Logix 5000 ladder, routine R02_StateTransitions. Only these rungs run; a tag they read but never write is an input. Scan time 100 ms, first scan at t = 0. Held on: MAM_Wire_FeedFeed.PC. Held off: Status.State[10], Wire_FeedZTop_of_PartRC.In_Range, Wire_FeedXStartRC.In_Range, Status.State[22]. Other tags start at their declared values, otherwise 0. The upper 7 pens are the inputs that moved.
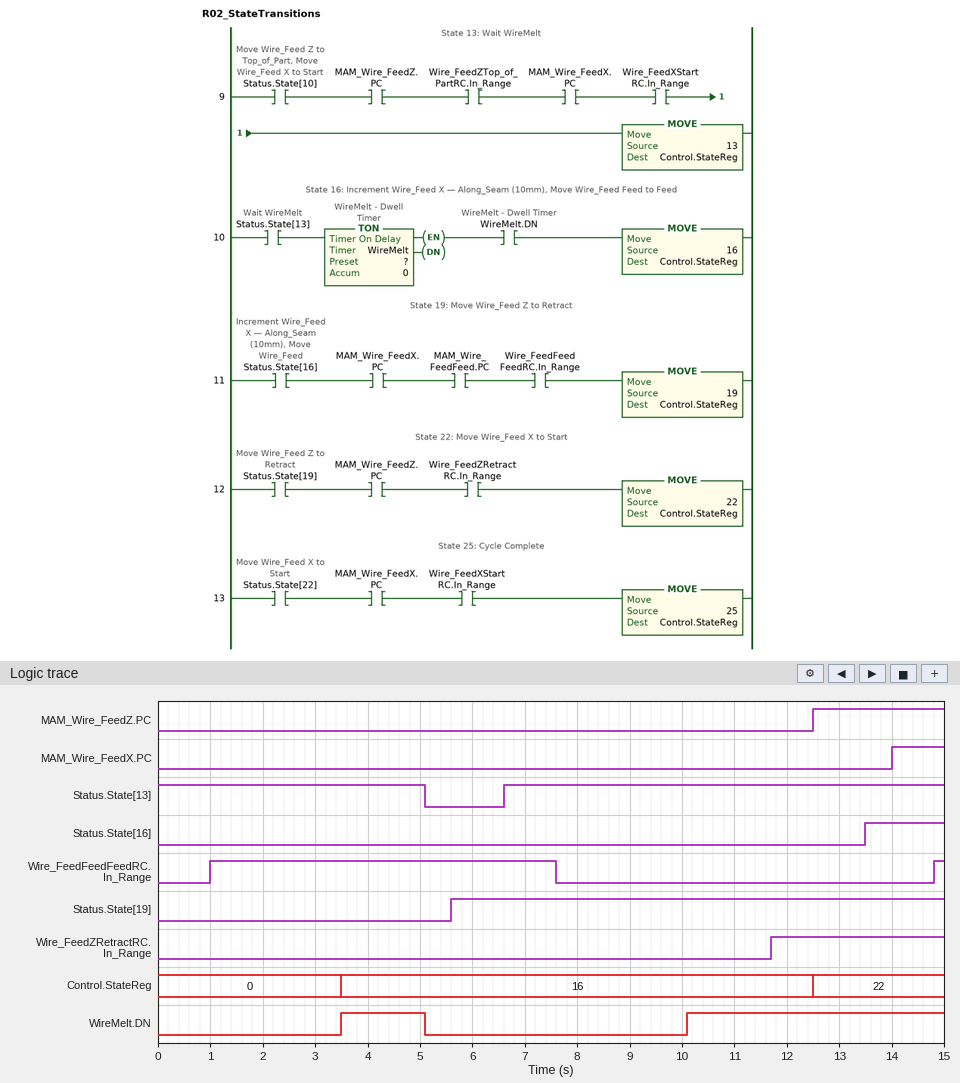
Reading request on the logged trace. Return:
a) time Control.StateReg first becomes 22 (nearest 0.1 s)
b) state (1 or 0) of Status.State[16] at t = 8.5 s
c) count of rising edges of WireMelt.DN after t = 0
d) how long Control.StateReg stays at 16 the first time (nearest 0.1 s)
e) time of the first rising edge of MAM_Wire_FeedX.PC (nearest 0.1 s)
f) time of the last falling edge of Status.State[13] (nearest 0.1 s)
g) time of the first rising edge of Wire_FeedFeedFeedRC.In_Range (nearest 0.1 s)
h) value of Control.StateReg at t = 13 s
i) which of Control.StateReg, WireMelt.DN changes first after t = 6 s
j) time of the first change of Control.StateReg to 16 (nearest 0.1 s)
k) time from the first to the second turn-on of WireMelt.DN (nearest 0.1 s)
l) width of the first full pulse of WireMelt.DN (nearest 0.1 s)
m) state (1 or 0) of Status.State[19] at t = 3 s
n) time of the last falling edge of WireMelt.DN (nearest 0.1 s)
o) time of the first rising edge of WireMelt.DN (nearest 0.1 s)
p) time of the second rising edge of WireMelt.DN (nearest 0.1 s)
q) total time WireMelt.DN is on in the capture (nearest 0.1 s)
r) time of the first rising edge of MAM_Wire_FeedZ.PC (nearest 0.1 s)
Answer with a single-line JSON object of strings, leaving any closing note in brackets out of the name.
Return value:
{"time Control.StateReg first becomes 22": "12.5 s", "state (1 or 0) of Status.State[16] at t = 8.5 s": "0", "count of rising edges of WireMelt.DN after t = 0": "2", "how long Control.StateReg stays at 16 the first time": "9.0 s", "time of the first rising edge of MAM_Wire_FeedX.PC": "14.0 s", "time of the last falling edge of Status.State[13]": "5.1 s", "time of the first rising edge of Wire_FeedFeedFeedRC.In_Range": "1.0 s", "value of Control.StateReg at t = 13 s": "22", "which of Control.StateReg, WireMelt.DN changes first after t = 6 s": "WireMelt.DN", "time of the first change of Control.StateReg to 16": "3.5 s", "time from the first to the second turn-on of WireMelt.DN": "6.6 s", "width of the first full pulse of WireMelt.DN": "1.6 s", "state (1 or 0) of Status.State[19] at t = 3 s": "0", "time of the last falling edge of WireMelt.DN": "5.1 s", "time of the first rising edge of WireMelt.DN": "3.5 s", "time of the second rising edge of WireMelt.DN": "10.1 s", "total time WireMelt.DN is on in the capture": "6.5 s", "time of the first rising edge of MAM_Wire_FeedZ.PC": "12.5 s"}
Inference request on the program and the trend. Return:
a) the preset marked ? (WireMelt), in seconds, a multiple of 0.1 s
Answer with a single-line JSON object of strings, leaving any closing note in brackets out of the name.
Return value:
{"the preset marked ? (WireMelt), in seconds, a multiple of 0.1 s": "3.5 s"}
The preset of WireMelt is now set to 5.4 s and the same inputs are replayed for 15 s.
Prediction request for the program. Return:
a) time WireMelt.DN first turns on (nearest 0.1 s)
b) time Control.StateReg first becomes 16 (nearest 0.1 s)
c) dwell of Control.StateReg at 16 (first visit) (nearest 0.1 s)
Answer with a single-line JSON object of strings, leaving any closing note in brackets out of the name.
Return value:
{"time WireMelt.DN first turns on": "12.0 s", "time Control.StateReg first becomes 16": "12.0 s", "dwell of Control.StateReg at 16 (first visit)": "0.5 s"}
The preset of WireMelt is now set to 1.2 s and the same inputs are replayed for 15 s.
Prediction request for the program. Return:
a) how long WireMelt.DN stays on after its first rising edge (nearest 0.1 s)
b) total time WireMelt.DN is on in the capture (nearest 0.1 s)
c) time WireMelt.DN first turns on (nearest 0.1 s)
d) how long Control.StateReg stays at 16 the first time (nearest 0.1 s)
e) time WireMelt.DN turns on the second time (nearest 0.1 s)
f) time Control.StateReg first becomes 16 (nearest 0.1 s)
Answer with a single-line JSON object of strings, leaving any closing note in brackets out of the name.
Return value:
{"how long WireMelt.DN stays on after its first rising edge": "3.9 s", "total time WireMelt.DN is on in the capture": "11.1 s", "time WireMelt.DN first turns on": "1.2 s", "how long Control.StateReg stays at 16 the first time": "11.3 s", "time WireMelt.DN turns on the second time": "7.8 s", "time Control.StateReg first becomes 16": "1.2 s"}
